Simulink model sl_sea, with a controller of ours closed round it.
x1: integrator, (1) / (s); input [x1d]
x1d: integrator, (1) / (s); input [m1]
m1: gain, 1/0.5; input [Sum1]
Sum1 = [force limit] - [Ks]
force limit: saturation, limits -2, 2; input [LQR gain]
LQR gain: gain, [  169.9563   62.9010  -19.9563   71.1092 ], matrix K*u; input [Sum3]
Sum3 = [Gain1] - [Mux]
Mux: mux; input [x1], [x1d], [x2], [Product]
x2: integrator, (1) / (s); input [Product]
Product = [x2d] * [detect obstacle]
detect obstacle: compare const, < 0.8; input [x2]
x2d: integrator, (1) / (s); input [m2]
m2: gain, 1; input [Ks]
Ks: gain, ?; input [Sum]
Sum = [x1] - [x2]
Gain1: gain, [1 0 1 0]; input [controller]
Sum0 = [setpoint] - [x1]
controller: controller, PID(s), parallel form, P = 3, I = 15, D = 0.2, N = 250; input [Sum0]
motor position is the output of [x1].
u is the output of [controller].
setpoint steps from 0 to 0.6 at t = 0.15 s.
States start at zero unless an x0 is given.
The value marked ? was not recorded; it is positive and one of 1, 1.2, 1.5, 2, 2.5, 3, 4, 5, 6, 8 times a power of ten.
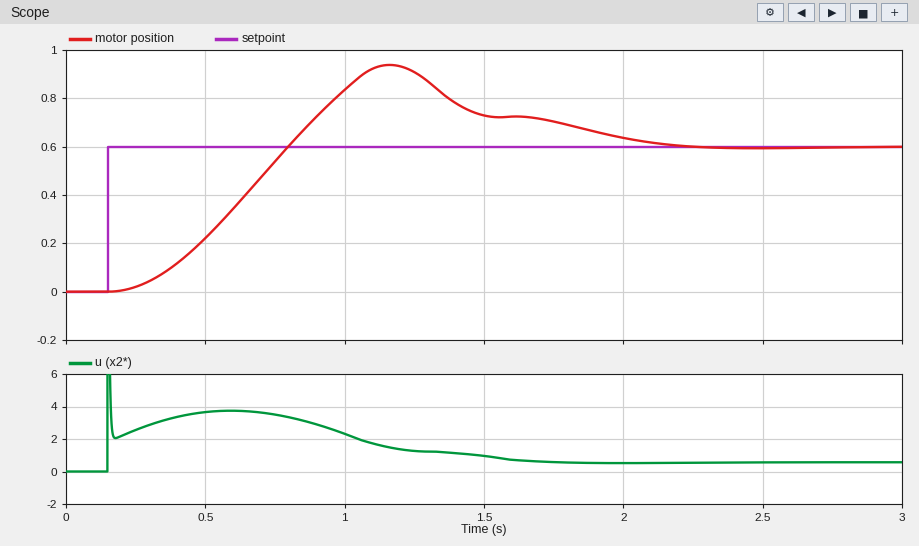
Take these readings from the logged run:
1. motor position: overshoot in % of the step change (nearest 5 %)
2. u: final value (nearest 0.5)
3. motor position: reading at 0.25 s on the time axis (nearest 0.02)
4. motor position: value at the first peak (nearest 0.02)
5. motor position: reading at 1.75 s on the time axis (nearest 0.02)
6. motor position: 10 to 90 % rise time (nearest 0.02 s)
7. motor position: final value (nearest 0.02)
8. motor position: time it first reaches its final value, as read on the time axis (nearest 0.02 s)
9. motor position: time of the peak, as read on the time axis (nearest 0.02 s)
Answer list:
55 %
0.5
0.02
0.94
0.70
0.42 s
0.60
0.80 s
1.16 s
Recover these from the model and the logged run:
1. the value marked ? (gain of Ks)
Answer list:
5
